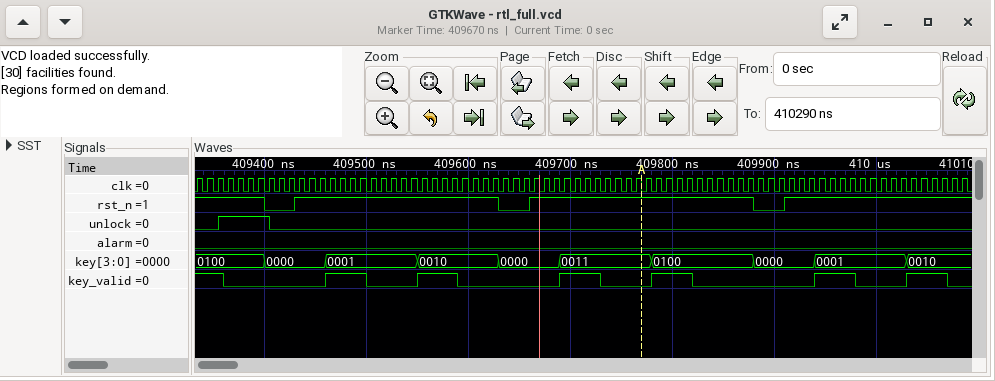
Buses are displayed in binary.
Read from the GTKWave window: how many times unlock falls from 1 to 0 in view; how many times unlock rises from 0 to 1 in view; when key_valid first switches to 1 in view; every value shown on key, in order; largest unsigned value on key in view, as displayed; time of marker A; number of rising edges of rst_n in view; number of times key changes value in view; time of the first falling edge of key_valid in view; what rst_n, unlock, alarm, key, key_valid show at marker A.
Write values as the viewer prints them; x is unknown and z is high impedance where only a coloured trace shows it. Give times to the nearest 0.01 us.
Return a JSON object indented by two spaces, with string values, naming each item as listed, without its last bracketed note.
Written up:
{
  "how many times unlock falls from 1 to 0 in view": "1",
  "how many times unlock rises from 0 to 1 in view": "1",
  "when key_valid first switches to 1 in view": "409.46 us",
  "every value shown on key, in order": "0100, 0000, 0001, 0010, 0000, 0011, 0100, 0000, 0001, 0010",
  "largest unsigned value on key in view, as displayed": "0100",
  "time of marker A": "409.77 us",
  "number of rising edges of rst_n in view": "3",
  "number of times key changes value in view": "9",
  "time of the first falling edge of key_valid in view": "409.36 us",
  "what rst_n, unlock, alarm, key, key_valid show at marker A": "rst_n=1, unlock=0, alarm=0, key=0011, key_valid=0"
}
